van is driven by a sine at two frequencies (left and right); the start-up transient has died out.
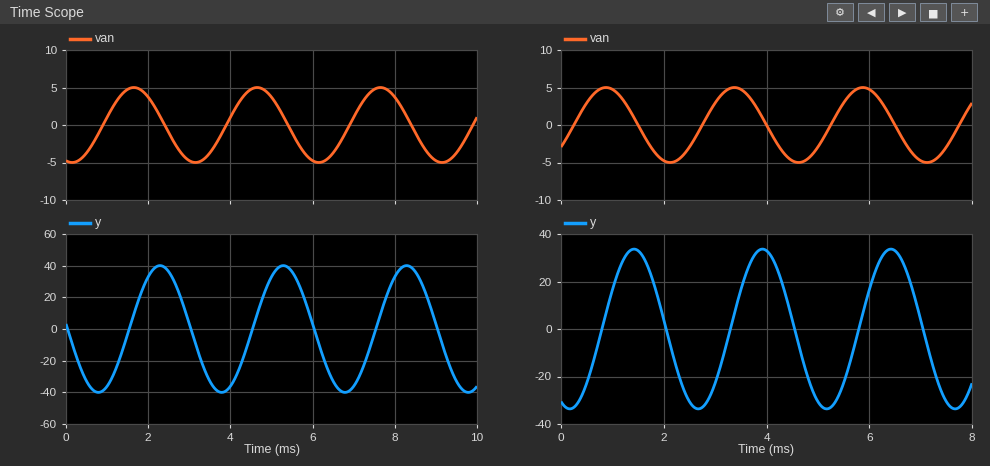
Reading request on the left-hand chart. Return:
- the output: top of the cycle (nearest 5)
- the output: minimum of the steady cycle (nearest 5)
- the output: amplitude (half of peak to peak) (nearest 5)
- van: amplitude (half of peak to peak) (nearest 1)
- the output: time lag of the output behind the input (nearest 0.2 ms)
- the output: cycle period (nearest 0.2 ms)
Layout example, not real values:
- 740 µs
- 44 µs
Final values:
- 40
- -40
- 40
- 5
- 0.6 ms
- 3.0 ms
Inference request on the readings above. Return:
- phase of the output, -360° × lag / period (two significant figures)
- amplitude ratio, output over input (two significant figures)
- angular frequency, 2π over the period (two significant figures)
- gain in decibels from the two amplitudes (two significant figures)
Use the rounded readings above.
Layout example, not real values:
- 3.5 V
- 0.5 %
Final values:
- -72°
- 8.0
- 2.1 rad/ms
- 18 dB
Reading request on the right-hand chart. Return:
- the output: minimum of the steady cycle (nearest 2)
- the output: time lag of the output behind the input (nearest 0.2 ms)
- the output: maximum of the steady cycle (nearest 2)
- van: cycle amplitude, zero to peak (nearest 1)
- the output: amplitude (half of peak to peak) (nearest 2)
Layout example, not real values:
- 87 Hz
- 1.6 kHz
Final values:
- -34
- 0.6 ms
- 34
- 5
- 34
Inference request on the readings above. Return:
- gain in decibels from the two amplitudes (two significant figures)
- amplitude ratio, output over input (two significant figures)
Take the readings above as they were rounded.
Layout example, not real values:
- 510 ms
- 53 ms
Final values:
- 17 dB
- 6.8
